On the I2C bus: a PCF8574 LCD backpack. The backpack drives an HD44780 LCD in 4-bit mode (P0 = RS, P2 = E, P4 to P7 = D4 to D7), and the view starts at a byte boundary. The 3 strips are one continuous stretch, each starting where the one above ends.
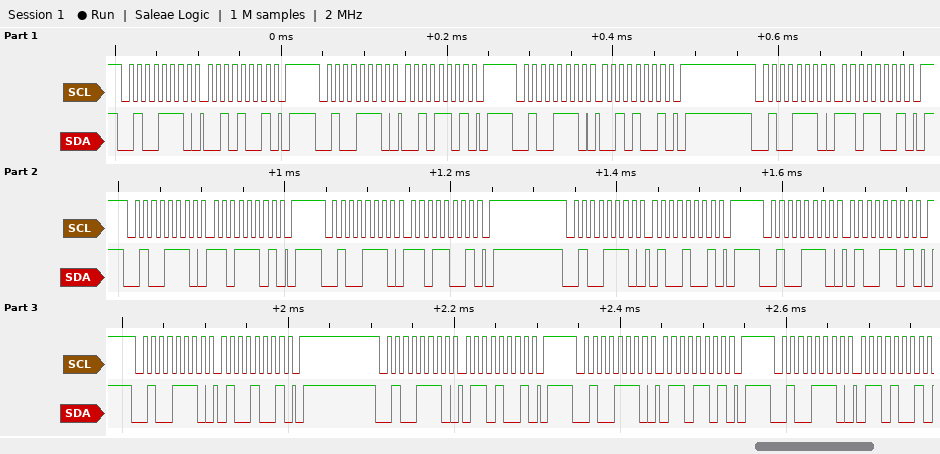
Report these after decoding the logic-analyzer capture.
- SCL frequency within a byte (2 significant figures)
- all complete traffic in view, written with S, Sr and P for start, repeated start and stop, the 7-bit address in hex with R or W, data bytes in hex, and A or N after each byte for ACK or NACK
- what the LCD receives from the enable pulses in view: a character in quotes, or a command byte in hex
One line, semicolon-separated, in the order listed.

100 kHz; S 27W A 29 A P S 27W A 2D A P S 27W A 29 A P S 27W A D9 A P S 27W A DD A P S 27W A D9 A P S 27W A 49 A P S 27W A 4D A P S 27W A 49 A P S 27W A 69 A P S 27W A 6D A P S 27W A 69 A; '-' 'F'
